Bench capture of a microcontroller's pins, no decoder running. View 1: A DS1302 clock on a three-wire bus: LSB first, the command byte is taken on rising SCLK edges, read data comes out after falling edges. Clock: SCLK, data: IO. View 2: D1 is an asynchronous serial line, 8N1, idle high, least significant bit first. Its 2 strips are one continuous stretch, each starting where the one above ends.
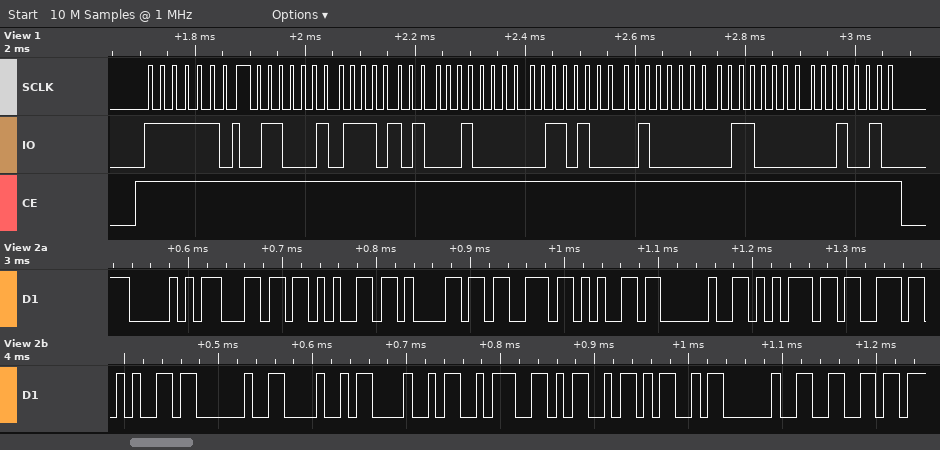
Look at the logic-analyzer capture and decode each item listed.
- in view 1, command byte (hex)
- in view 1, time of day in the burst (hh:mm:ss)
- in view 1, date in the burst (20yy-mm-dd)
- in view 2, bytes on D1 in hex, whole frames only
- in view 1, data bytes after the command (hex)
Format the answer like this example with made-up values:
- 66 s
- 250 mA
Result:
- 0xBF
- 04:57:46
- 2024-02-16
- 50 6C 65 61 73 65 20 75 73 65 20 48 48 3A 4D 4D 20 66
- 46 57 04 16 02 06 24
